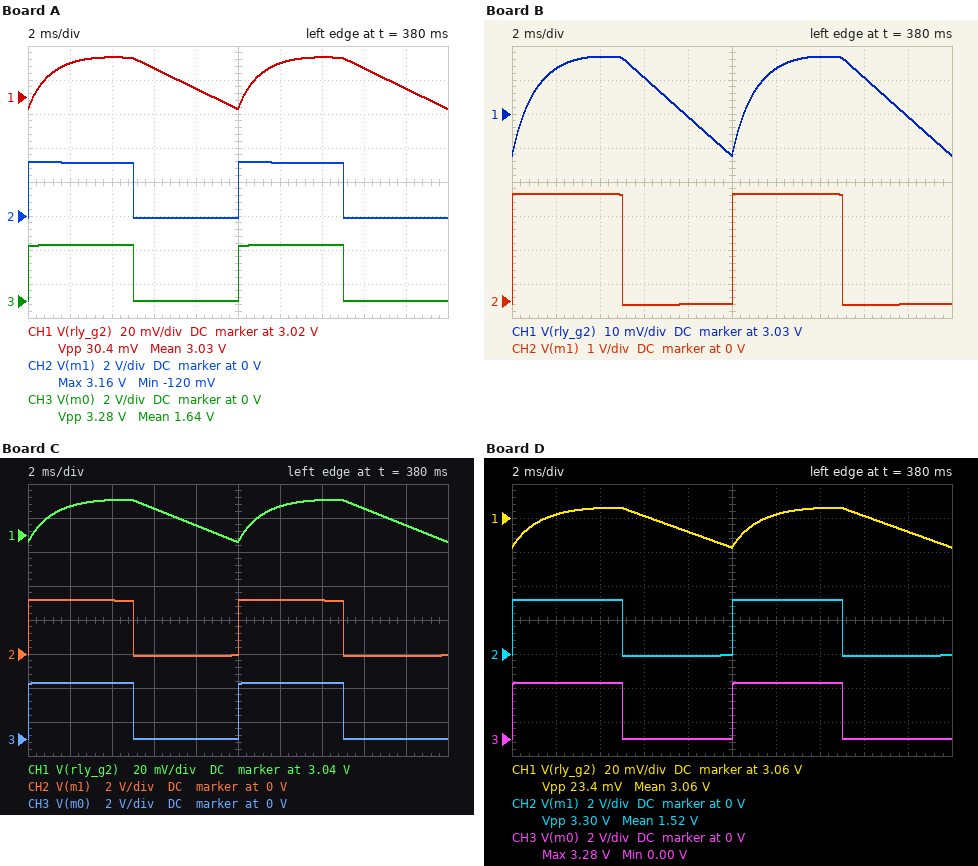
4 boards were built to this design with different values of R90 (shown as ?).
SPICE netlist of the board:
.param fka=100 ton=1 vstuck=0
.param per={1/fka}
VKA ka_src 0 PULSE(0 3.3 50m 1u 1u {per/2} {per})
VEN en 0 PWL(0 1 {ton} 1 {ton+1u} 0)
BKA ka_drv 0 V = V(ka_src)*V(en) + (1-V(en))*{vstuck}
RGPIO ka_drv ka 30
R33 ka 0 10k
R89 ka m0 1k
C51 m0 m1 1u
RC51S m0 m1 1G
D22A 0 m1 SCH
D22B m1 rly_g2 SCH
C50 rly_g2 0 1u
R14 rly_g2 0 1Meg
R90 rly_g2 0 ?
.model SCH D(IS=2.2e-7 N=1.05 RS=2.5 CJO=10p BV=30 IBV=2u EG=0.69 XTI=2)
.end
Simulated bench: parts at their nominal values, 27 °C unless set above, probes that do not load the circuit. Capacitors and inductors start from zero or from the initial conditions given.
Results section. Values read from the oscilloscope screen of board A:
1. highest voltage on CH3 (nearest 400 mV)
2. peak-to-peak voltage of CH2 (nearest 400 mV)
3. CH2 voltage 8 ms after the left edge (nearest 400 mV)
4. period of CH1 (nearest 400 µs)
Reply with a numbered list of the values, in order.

1. 3.2 V
2. 3.2 V
3. 0 V
4. 10.0 ms
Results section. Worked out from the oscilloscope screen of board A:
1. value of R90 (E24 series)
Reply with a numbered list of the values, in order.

1. 1.1 MΩ
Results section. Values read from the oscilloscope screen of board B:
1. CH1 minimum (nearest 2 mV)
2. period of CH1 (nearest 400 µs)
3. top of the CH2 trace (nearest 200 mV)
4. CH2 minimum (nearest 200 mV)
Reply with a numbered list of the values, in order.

1. 3.018 V
2. 10.0 ms
3. 3.2 V
4. -200 mV
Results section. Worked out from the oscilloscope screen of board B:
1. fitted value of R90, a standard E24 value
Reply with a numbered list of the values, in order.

1. 1.2 MΩ
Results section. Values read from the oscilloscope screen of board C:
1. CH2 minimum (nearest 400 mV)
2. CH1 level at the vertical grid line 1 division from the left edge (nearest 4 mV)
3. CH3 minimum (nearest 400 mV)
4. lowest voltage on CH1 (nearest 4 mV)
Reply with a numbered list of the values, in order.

1. 0 V
2. 3.056 V
3. 0 V
4. 3.036 V
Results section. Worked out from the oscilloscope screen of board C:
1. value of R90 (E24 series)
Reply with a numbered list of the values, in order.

1. 1.8 MΩ
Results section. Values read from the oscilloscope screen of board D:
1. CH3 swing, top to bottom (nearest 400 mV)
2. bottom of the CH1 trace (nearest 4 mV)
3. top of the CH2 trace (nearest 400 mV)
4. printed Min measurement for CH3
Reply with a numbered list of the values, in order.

1. 3.2 V
2. 3.044 V
3. 3.2 V
4. 0.00 V
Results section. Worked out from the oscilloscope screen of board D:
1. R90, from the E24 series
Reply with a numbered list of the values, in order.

1. 2.2 MΩ
